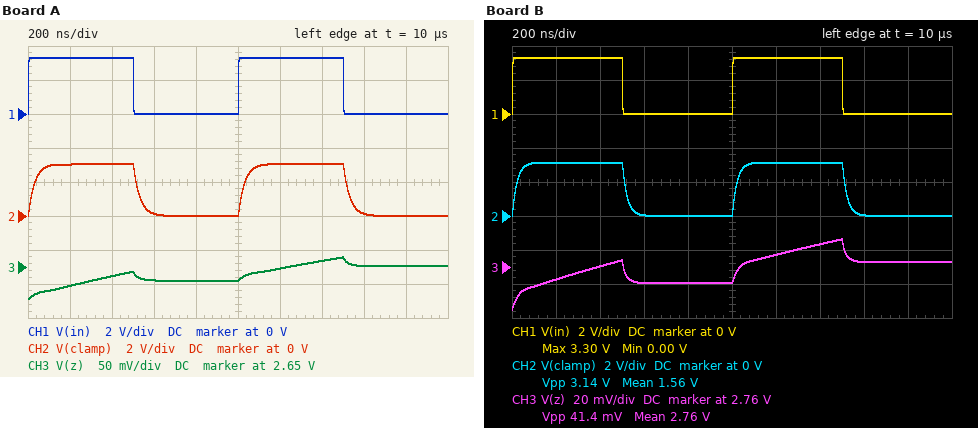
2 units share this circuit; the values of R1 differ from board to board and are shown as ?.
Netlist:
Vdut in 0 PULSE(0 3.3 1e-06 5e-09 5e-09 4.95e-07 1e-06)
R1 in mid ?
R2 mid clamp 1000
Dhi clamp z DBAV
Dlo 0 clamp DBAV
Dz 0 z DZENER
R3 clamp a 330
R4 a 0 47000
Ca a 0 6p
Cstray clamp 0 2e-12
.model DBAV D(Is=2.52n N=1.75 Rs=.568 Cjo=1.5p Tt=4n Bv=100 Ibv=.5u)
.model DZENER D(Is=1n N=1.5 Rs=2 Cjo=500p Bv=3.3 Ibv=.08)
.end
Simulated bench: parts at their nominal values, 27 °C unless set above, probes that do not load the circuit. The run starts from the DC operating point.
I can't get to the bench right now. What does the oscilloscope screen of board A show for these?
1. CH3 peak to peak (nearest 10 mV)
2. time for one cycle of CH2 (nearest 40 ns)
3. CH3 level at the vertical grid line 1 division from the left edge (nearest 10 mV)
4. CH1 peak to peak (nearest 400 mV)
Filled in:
60 mV
1.00 µs
2.62 V
3.2 V
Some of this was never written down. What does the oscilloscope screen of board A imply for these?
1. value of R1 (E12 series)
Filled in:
2.2 kΩ
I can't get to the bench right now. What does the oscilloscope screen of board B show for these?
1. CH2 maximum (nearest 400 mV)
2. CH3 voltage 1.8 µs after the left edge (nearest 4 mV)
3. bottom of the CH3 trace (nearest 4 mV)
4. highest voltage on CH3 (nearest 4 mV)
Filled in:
3.2 V
2.764 V
2.736 V
2.776 V
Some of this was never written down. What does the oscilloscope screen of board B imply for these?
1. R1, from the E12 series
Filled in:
1.2 kΩ
